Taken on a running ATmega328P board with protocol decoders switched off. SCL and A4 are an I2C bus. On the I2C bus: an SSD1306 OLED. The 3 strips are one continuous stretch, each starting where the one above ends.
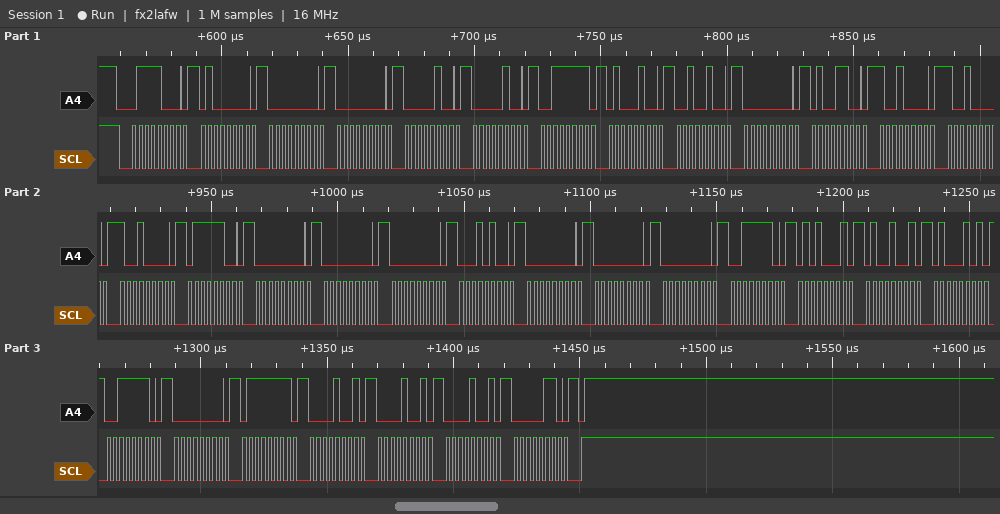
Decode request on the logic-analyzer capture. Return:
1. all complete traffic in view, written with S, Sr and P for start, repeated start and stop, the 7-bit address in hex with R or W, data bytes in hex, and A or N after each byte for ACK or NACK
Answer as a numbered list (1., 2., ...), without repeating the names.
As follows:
1. S 3CW A 40 A 00 A 00 A 04 A 04 A 3F A 44 A 24 A 00 A 4C A 90 A 90 A 90 A 7C A 00 A 00 A 00 A 14 A 00 A 00 A 00 A 3E A 51 A 49 A 45 A 3E A 00 A 7F A 09 A 09 A 09 A 06 A P
